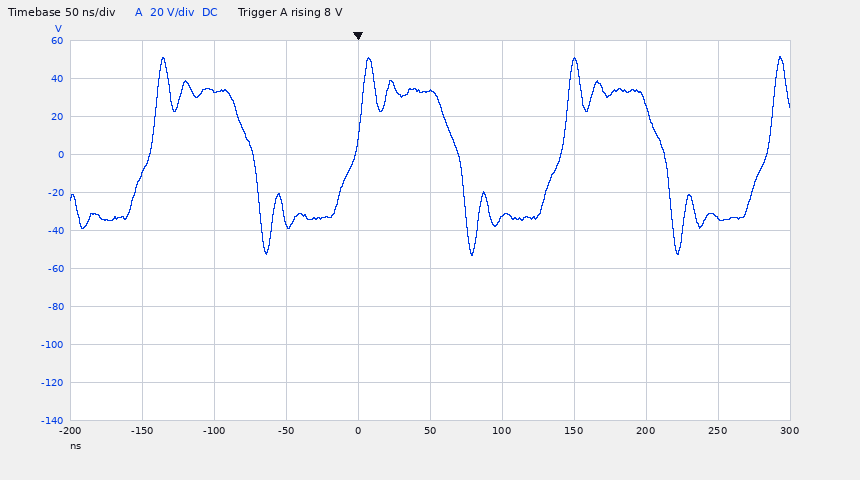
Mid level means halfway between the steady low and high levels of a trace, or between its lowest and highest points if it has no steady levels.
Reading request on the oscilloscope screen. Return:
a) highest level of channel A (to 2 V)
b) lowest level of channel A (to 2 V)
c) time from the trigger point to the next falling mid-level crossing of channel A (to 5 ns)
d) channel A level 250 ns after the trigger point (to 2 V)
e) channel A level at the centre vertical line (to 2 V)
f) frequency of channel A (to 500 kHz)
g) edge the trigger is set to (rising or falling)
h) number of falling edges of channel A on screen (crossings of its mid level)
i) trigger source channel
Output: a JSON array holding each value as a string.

["52 V", "-54 V", "70 ns", "-34 V", "34 V", "7.0 MHz", "rising", "3", "channel A"]
